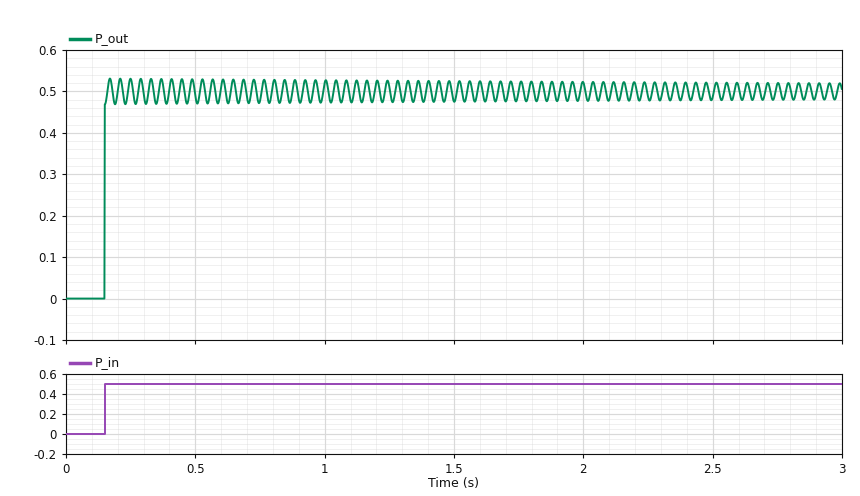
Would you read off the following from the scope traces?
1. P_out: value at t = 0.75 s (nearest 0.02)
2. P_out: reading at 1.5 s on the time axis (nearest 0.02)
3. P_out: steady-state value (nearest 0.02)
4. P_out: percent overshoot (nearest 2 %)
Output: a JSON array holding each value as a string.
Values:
["0.48", "0.48", "0.50", "6 %"]
